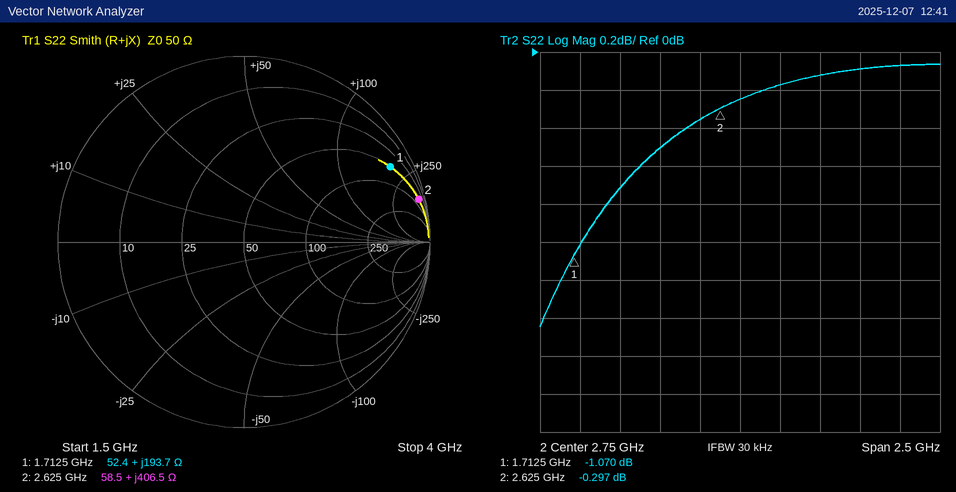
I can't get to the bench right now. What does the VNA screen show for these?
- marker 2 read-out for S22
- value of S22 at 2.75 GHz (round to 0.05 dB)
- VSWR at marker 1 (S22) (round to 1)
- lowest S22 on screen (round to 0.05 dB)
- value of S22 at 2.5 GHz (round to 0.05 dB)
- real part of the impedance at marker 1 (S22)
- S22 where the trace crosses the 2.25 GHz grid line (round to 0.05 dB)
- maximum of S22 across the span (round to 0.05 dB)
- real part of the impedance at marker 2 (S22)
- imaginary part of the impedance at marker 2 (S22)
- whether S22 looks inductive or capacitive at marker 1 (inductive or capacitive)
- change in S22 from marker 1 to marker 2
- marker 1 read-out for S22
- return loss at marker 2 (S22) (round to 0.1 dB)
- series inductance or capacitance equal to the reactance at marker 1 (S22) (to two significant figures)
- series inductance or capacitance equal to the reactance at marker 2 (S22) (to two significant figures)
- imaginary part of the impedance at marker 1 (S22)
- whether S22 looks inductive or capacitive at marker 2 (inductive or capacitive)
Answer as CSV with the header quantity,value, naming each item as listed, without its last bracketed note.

quantity,value
marker 2 read-out for S22,-0.297 dB
value of S22 at 2.75 GHz,-0.25 dB
VSWR at marker 1 (S22),16
lowest S22 on screen,-1.45 dB
value of S22 at 2.5 GHz,-0.35 dB
real part of the impedance at marker 1,52.4 Ω
S22 where the trace crosses the 2.25 GHz grid line,-0.50 dB
maximum of S22 across the span,-0.05 dB
real part of the impedance at marker 2,58.5 Ω
imaginary part of the impedance at marker 2,+406.5 Ω
whether S22 looks inductive or capacitive at marker 1,inductive
change in S22 from marker 1 to marker 2,0.773 dB
marker 1 read-out for S22,-1.070 dB
return loss at marker 2 (S22),0.3 dB
series inductance or capacitance equal to the reactance at marker 1 (S22),18 nH
series inductance or capacitance equal to the reactance at marker 2 (S22),25 nH
imaginary part of the impedance at marker 1,+193.7 Ω
whether S22 looks inductive or capacitive at marker 2,inductive
